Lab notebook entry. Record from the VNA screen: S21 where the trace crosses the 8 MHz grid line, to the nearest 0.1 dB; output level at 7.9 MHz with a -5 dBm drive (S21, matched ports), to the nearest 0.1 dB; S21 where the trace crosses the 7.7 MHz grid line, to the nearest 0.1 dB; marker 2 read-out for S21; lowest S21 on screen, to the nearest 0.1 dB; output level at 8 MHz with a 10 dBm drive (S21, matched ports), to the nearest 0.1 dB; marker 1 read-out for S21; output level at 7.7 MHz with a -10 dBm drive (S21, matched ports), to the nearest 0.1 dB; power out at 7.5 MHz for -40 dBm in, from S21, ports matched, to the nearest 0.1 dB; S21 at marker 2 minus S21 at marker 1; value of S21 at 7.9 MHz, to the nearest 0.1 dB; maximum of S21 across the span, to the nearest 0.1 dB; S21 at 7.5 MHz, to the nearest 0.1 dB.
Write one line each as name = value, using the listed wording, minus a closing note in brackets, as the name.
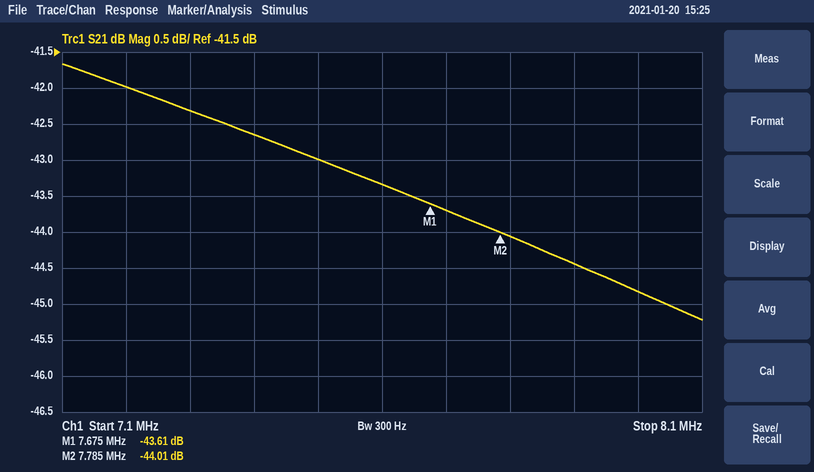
S21 where the trace crosses the 8 MHz grid line, to the nearest 0.1 dB = -44.8 dB
output level at 7.9 MHz with a -5 dBm drive (S21, matched ports), to the nearest 0.1 dB = -49.4 dBm
S21 where the trace crosses the 7.7 MHz grid line, to the nearest 0.1 dB = -43.7 dB
marker 2 read-out for S21 = -44.01 dB
lowest S21 on screen, to the nearest 0.1 dB = -45.2 dB
output level at 8 MHz with a 10 dBm drive (S21, matched ports), to the nearest 0.1 dB = -34.8 dBm
marker 1 read-out for S21 = -43.61 dB
output level at 7.7 MHz with a -10 dBm drive (S21, matched ports), to the nearest 0.1 dB = -53.7 dBm
power out at 7.5 MHz for -40 dBm in, from S21, ports matched, to the nearest 0.1 dB = -83.0 dBm
S21 at marker 2 minus S21 at marker 1 = -0.40 dB
value of S21 at 7.9 MHz, to the nearest 0.1 dB = -44.4 dB
maximum of S21 across the span, to the nearest 0.1 dB = -41.7 dB
S21 at 7.5 MHz, to the nearest 0.1 dB = -43.0 dB
